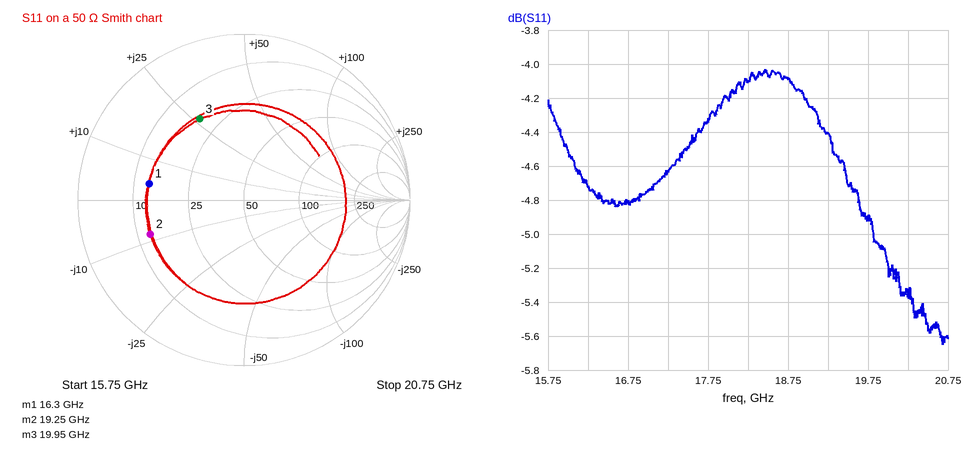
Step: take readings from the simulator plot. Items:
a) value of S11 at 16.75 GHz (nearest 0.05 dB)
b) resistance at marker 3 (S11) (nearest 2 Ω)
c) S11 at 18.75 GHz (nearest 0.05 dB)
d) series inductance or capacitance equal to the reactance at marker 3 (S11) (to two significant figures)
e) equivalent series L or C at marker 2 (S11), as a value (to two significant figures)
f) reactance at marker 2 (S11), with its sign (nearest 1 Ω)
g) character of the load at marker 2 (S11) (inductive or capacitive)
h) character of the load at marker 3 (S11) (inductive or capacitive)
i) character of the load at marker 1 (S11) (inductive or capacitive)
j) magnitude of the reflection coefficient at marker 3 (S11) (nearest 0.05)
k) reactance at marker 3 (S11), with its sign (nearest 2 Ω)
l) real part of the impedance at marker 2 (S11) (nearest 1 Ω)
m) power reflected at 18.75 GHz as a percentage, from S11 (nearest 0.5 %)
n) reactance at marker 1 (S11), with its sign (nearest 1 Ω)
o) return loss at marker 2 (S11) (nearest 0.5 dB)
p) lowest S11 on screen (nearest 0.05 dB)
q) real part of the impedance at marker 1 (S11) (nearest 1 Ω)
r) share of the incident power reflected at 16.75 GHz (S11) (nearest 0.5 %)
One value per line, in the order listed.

-4.80 dB
18 Ω
-4.10 dB
210 pH
1.0 pF
-8 Ω
capacitive
inductive
inductive
0.55
+26 Ω
13 Ω
39.0 %
+4 Ω
4.5 dB
-5.65 dB
13 Ω
33.0 %
